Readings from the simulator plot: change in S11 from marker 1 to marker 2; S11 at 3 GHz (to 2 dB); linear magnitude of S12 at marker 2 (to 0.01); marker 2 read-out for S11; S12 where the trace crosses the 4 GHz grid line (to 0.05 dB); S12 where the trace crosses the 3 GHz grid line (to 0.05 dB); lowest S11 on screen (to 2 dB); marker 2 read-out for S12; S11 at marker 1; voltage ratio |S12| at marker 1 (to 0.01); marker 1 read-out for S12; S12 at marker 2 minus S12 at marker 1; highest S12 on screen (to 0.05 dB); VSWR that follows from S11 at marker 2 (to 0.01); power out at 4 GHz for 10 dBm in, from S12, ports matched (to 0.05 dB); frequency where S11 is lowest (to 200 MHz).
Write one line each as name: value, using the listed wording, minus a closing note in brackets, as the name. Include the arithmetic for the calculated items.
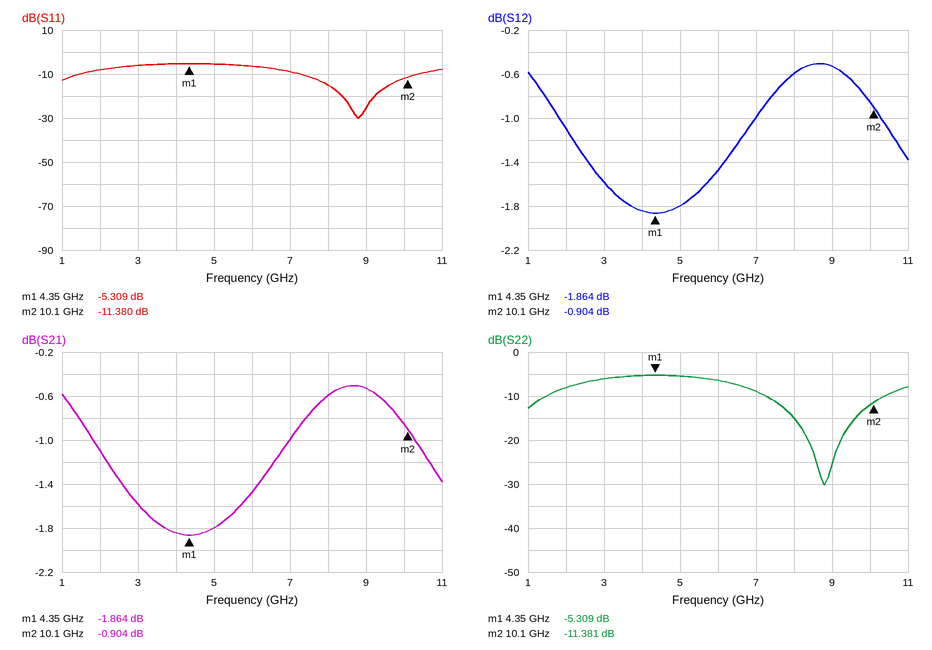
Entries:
change in S11 from marker 1 to marker 2: -11.38 − (-5.309) = -6.071 dB
S11 at 3 GHz: -6 dB
linear magnitude of S12 at marker 2: 10^(-0.904/20) ≈ 0.90
marker 2 read-out for S11: -11.380 dB
S12 where the trace crosses the 4 GHz grid line: -1.85 dB
S12 where the trace crosses the 3 GHz grid line: -1.60 dB
lowest S11 on screen: -30 dB
marker 2 read-out for S12: -0.904 dB
S11 at marker 1: -5.309 dB
voltage ratio |S12| at marker 1: 10^(-1.864/20) ≈ 0.81
marker 1 read-out for S12: -1.864 dB
S12 at marker 2 minus S12 at marker 1: -0.904 − (-1.864) = 0.960 dB
highest S12 on screen: -0.50 dB
VSWR that follows from S11 at marker 2: (1 + 0.2698)/(1 − 0.2698) ≈ 1.74
power out at 4 GHz for 10 dBm in, from S12, ports matched: 10 dBm + (-1.85 dB) = 8.15 dBm
frequency where S11 is lowest: 8.8 GHz
